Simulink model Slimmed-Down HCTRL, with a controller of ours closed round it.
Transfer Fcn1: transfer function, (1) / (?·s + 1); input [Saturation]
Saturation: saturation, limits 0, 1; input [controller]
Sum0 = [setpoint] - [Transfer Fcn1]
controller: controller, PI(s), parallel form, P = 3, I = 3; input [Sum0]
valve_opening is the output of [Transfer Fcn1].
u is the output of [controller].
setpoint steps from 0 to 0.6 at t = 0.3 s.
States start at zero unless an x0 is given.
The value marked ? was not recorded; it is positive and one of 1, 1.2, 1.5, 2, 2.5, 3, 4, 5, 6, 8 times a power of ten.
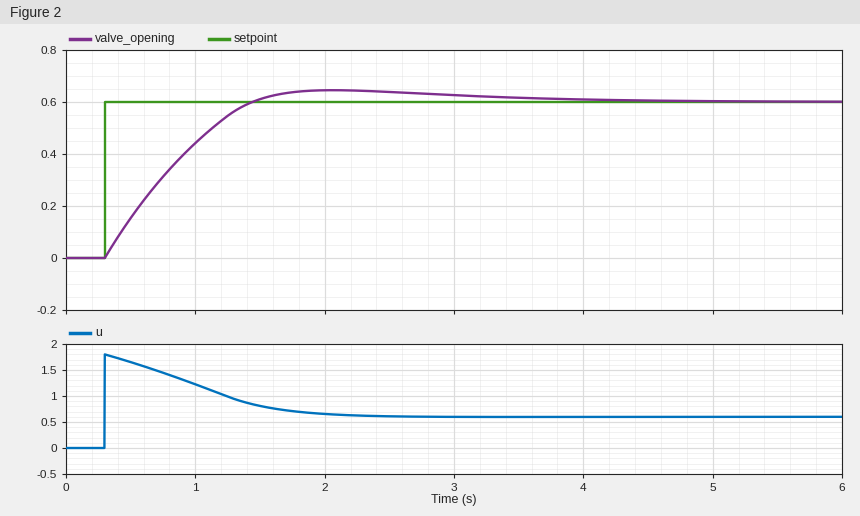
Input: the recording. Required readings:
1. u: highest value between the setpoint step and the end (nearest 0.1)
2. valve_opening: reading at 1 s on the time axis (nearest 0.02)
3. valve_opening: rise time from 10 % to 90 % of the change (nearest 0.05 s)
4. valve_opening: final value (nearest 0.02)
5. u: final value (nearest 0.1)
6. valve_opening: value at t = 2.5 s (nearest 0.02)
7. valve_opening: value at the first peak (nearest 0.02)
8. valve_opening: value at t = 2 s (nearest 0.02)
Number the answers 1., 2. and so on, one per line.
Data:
1. 1.8
2. 0.44
3. 0.85 s
4. 0.60
5. 0.6
6. 0.64
7. 0.64
8. 0.64
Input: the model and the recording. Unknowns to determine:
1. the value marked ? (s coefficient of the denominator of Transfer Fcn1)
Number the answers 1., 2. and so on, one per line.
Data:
1. 1.2
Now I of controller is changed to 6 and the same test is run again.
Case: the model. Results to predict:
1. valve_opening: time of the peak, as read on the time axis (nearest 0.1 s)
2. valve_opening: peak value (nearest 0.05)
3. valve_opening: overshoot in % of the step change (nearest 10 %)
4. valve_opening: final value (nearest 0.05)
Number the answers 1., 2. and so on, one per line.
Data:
1. 2.1 s
2. 0.75
3. 30 %
4. 0.60
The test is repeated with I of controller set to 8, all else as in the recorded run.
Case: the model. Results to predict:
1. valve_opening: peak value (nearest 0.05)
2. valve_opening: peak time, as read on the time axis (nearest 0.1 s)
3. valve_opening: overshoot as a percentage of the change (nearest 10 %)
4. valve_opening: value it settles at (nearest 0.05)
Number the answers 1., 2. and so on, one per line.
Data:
1. 0.80
2. 2.3 s
3. 30 %
4. 0.60
